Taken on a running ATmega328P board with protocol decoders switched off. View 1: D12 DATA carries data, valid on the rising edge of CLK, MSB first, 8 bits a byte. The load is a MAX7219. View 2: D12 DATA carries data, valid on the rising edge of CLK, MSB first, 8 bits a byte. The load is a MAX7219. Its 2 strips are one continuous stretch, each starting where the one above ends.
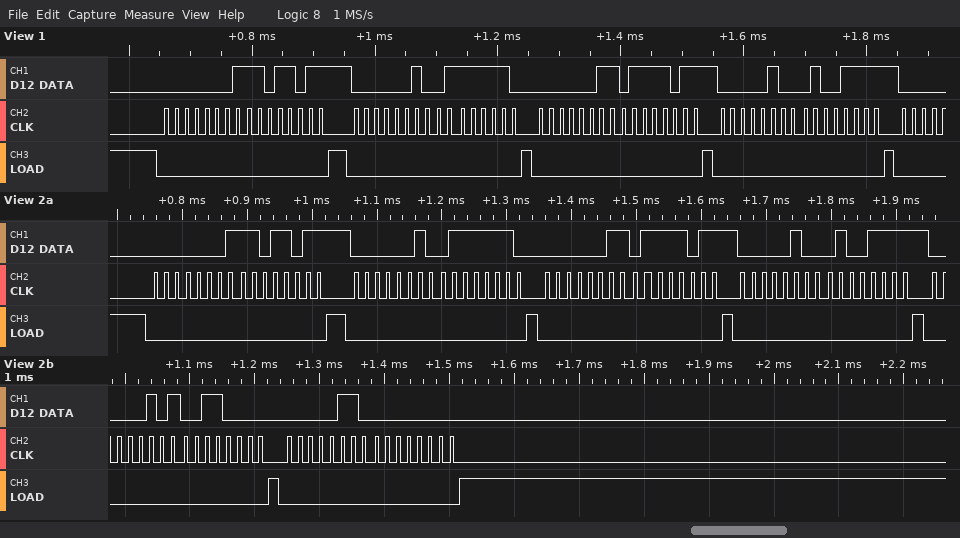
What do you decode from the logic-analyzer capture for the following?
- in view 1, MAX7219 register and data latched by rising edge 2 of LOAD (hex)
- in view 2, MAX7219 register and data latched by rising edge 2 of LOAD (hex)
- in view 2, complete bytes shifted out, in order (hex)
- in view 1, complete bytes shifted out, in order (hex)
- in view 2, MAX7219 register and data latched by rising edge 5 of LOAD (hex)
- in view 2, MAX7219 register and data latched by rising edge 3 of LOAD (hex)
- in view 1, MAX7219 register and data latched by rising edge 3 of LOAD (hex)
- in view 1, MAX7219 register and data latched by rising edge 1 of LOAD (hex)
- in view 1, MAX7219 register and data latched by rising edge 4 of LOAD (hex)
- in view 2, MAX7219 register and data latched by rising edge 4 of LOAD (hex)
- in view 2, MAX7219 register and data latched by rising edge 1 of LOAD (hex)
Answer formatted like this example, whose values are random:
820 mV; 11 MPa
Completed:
register 0x2, data 0x7E; register 0x2, data 0x7E; 0x01 0xDB 0x02 0x7E 0x03 0x7B 0x04 0x4F 0x05 0x30 0x06 0x00; 01 DB 02 7E 03 7B 04 4F; register 0x5, data 0x30; register 0x3, data 0x7B; register 0x3, data 0x7B; register 0x1, data 0xDB; register 0x4, data 0x4F; register 0x4, data 0x4F; register 0x1, data 0xDB
